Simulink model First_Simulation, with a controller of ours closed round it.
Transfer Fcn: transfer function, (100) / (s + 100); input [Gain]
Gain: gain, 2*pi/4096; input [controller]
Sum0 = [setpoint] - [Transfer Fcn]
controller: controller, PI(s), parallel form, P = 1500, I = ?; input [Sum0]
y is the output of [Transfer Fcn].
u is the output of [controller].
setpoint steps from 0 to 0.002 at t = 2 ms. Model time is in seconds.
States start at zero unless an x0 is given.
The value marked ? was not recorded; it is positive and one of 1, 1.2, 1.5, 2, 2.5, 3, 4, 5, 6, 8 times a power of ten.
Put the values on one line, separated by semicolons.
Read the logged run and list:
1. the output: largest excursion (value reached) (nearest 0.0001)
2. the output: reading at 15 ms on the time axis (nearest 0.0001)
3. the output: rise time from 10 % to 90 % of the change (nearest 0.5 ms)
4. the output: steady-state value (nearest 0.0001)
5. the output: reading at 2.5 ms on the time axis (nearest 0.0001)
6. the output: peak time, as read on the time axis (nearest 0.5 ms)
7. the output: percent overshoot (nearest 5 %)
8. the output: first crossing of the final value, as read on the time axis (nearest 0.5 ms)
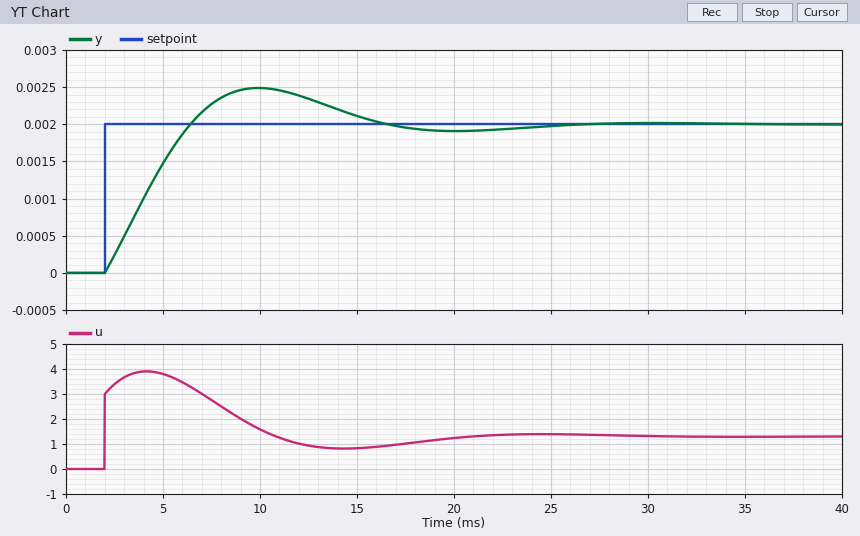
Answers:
0.0025; 0.0021; 3.5 ms; 0.0020; 0.0002; 10.0 ms; 25 %; 6.5 ms
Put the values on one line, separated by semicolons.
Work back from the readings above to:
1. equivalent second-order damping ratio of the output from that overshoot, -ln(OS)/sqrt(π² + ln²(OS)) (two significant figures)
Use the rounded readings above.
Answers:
0.40
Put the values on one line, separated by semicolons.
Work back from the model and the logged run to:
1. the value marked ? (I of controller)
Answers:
800000
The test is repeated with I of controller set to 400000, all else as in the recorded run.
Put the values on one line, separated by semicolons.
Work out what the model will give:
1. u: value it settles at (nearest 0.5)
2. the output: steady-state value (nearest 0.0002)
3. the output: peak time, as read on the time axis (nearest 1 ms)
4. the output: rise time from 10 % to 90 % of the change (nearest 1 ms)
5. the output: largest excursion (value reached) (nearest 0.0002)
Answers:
1.5; 0.0020; 13 ms; 5 ms; 0.0022
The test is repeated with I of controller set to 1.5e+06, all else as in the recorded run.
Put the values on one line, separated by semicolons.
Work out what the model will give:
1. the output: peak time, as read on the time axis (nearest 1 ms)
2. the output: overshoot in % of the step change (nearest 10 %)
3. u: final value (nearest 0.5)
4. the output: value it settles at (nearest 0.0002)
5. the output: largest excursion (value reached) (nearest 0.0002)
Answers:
8 ms; 40 %; 1.5; 0.0020; 0.0028
